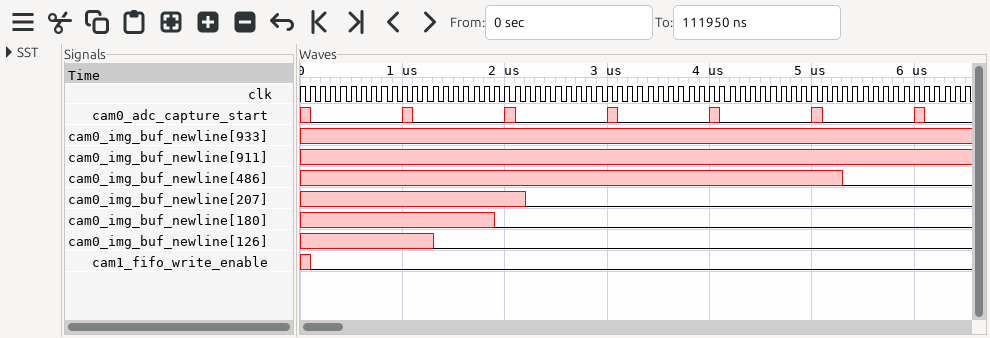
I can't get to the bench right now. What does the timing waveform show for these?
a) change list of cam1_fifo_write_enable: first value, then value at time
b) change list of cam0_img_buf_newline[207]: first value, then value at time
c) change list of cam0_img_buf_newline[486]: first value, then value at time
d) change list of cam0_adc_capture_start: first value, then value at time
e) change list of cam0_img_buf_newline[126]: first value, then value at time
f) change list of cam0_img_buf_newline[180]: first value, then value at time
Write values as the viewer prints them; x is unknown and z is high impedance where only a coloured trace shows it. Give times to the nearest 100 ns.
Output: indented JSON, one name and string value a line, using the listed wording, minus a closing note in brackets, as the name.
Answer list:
{
  "change list of cam1_fifo_write_enable: first value, then value at time": "x, 0 at 100 ns",
  "change list of cam0_img_buf_newline[207]: first value, then value at time": "x, 0 at 2200 ns",
  "change list of cam0_img_buf_newline[486]: first value, then value at time": "x, 0 at 5300 ns",
  "change list of cam0_adc_capture_start: first value, then value at time": "x, 0 at 100 ns, x at 1000 ns, 0 at 1100 ns, x at 2000 ns, 0 at 2100 ns, x at 3000 ns, 0 at 3100 ns, x at 4000 ns, 0 at 4100 ns, x at 5000 ns, 0 at 5100 ns, x at 6000 ns, 0 at 6100 ns",
  "change list of cam0_img_buf_newline[126]: first value, then value at time": "x, 0 at 1300 ns",
  "change list of cam0_img_buf_newline[180]: first value, then value at time": "x, 0 at 1900 ns"
}
